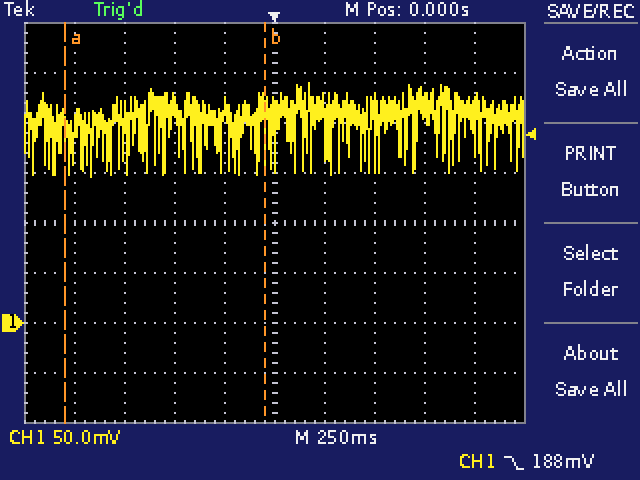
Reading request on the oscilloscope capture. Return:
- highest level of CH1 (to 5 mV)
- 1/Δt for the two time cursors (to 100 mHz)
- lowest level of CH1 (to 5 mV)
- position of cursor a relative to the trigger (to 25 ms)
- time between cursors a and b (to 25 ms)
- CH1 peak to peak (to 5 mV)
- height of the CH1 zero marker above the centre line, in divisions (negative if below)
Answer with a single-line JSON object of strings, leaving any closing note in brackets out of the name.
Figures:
{"highest level of CH1": "240 mV", "1/Δt for the two time cursors": "1.0 Hz", "lowest level of CH1": "145 mV", "position of cursor a relative to the trigger": "-1.050 s", "time between cursors a and b": "1.000 s", "CH1 peak to peak": "95 mV", "height of the CH1 zero marker above the centre line, in divisions": "-2.0 div"}
